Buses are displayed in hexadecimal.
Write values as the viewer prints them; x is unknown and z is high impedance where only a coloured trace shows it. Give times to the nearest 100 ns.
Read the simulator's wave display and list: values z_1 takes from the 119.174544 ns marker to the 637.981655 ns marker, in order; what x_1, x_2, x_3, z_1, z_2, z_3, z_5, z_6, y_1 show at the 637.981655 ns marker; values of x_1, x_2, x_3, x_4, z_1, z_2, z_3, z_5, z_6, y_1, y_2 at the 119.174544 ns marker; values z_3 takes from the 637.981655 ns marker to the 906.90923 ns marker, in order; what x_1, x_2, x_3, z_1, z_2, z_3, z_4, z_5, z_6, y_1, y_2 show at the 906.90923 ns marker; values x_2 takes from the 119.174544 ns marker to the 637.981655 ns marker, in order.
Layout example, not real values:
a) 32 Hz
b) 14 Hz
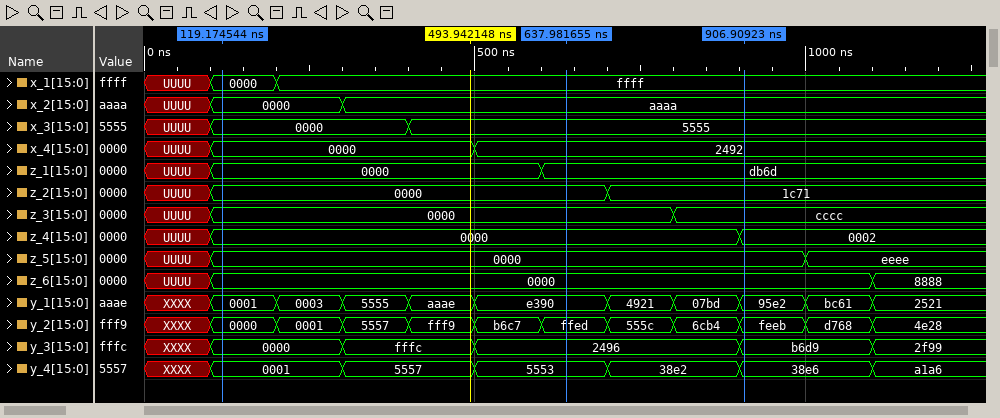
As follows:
a) 0000, db6d
b) x_1=ffff, x_2=aaaa, x_3=5555, z_1=db6d, z_2=0000, z_3=0000, z_5=0000, z_6=0000, y_1=e390
c) x_1=0000, x_2=0000, x_3=0000, x_4=0000, z_1=0000, z_2=0000, z_3=0000, z_5=0000, z_6=0000, y_1=0001, y_2=0000
d) 0000, cccc
e) x_1=ffff, x_2=aaaa, x_3=5555, z_1=db6d, z_2=1c71, z_3=cccc, z_4=0002, z_5=0000, z_6=0000, y_1=95e2, y_2=feeb
f) 0000, aaaa
